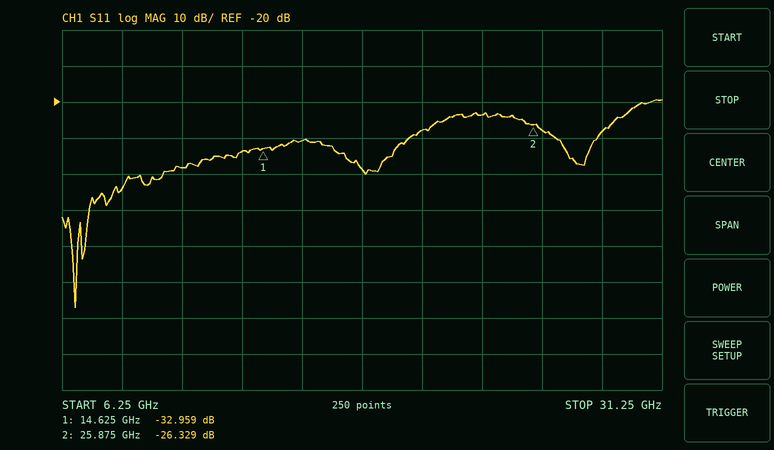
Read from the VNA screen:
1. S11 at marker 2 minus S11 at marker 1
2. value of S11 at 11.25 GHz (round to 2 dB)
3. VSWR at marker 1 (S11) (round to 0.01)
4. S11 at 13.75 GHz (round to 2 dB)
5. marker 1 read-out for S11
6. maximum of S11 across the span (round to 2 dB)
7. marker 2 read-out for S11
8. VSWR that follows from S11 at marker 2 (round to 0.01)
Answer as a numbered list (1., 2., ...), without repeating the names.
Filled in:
1. 6.630 dB
2. -38 dB
3. 1.05
4. -34 dB
5. -32.959 dB
6. -20 dB
7. -26.329 dB
8. 1.10
